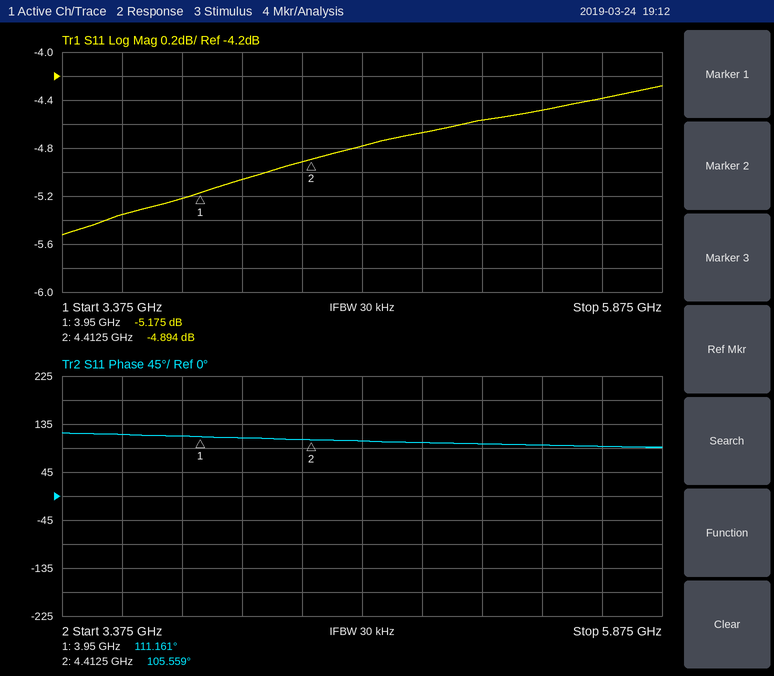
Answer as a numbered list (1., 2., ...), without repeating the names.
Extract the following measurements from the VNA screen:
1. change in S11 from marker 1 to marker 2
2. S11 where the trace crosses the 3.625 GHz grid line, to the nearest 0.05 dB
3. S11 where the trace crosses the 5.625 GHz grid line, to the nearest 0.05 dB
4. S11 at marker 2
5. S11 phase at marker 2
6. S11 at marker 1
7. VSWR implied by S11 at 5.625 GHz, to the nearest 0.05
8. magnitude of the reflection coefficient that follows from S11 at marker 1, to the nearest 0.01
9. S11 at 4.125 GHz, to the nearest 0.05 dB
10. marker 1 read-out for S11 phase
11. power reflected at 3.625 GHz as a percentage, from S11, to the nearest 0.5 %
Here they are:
1. 0.281 dB
2. -5.35 dB
3. -4.40 dB
4. -4.894 dB
5. 105.559°
6. -5.175 dB
7. 4.05
8. 0.55
9. -5.05 dB
10. 111.161°
11. 29.0 %
